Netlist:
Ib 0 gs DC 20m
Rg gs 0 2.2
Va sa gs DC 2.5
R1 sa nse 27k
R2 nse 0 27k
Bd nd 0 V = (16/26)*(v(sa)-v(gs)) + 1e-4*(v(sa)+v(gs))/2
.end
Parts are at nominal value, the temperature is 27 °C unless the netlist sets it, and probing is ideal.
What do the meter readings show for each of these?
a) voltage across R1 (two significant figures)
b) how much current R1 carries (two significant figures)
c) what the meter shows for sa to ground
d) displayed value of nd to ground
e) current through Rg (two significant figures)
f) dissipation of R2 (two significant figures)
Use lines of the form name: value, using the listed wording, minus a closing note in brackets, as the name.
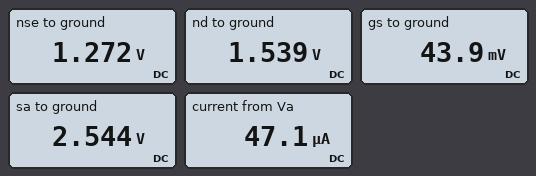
voltage across R1: 1.3 V
how much current R1 carries: 47 µA
what the meter shows for sa to ground: 2.544 V
displayed value of nd to ground: 1.539 V
current through Rg: 20 mA
dissipation of R2: 60 µW
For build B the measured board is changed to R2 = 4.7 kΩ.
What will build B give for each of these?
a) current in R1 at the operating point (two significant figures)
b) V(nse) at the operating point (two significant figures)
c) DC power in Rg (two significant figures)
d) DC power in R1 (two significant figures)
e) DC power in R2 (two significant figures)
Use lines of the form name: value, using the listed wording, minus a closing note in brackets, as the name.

current in R1 at the operating point: 80 µA
V(nse) at the operating point: 380 mV
DC power in Rg: 870 µW
DC power in R1: 170 µW
DC power in R2: 30 µW
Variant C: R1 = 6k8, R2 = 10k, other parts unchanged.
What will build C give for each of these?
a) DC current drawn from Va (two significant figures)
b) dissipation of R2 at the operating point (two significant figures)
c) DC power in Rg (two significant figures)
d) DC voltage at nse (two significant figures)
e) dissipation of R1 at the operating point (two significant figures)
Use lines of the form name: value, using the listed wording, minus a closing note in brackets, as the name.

DC current drawn from Va: 150 µA
dissipation of R2 at the operating point: 230 µW
DC power in Rg: 870 µW
DC voltage at nse: 1.5 V
dissipation of R1 at the operating point: 160 µW
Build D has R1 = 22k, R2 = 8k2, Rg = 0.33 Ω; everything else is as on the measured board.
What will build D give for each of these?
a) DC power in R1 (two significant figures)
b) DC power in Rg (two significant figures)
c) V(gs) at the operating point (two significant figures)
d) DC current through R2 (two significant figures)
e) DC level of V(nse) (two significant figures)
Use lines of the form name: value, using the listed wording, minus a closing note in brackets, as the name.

DC power in R1: 150 µW
DC power in Rg: 130 µW
V(gs) at the operating point: 6.6 mV
DC current through R2: 83 µA
DC level of V(nse): 680 mV
